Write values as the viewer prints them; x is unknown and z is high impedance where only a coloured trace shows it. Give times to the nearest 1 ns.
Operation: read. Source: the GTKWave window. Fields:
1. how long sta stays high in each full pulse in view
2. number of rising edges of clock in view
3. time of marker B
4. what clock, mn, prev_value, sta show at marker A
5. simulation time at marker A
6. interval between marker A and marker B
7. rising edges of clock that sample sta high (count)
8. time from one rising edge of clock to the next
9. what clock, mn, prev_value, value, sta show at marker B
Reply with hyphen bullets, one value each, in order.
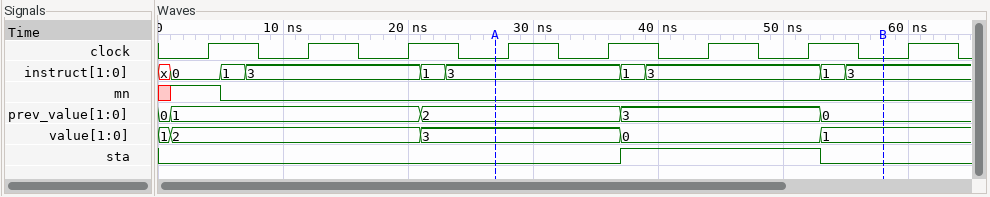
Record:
- 16 ns
- 8
- 58 ns
- clock=0, mn=0, prev_value=2, sta=0
- 27 ns
- 31 ns
- 2
- 8 ns
- clock=0, mn=0, prev_value=0, value=1, sta=0
